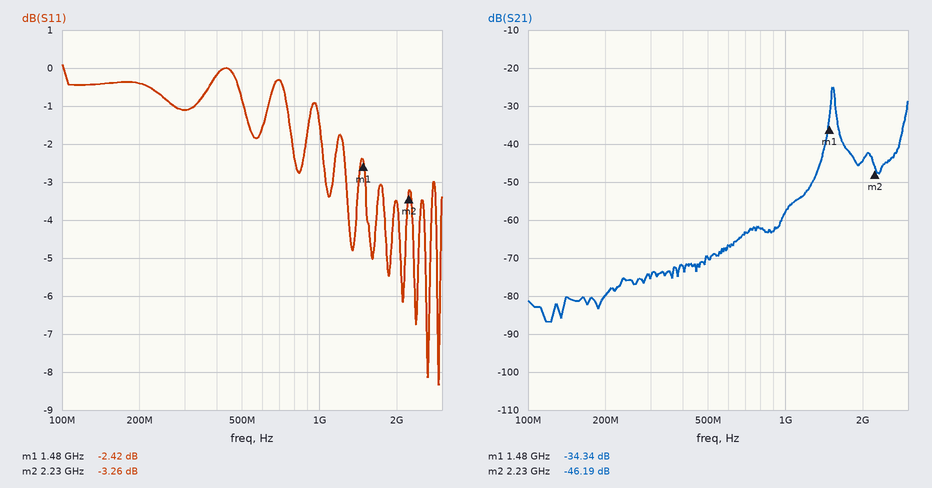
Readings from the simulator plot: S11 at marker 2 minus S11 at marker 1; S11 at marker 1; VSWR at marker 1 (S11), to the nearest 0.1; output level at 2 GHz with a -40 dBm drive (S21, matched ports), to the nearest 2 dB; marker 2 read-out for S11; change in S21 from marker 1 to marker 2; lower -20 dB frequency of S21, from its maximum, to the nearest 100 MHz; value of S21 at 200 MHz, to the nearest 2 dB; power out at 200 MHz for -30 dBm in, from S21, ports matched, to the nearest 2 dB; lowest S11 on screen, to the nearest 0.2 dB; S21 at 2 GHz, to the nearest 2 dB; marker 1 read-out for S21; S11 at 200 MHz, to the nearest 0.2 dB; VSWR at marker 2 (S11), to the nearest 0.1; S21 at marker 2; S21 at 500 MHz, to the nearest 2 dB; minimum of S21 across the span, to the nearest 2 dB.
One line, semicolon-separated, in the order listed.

-0.84 dB; -2.42 dB; 7.2; -84 dBm; -3.26 dB; -11.85 dB; 1.4 GHz; -80 dB; -110 dBm; -8.4 dB; -44 dB; -34.34 dB; -0.4 dB; 5.4; -46.19 dB; -70 dB; -86 dB
